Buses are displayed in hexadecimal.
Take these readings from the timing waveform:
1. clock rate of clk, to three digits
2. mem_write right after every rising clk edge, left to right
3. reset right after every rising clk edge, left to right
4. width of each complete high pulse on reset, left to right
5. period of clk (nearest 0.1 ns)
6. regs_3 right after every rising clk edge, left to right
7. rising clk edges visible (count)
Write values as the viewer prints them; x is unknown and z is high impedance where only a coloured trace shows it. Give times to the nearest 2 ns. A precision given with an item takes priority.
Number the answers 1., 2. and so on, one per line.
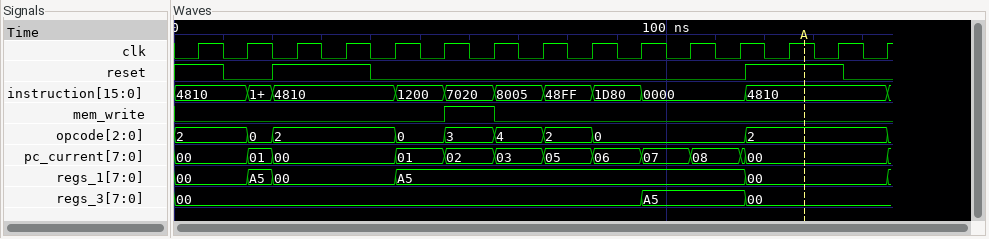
1. 100 MHz
2. 0 0 0 0 0 1 0 0 0 0 0 0 0 0 0
3. 1 0 1 1 0 0 0 0 0 0 0 0 1 1 0
4. 20 ns, 20 ns
5. 10 ns
6. 00, 00, 00, 00, 00, 00, 00, 00, 00, A5, A5, A5, 00, 00, 00
7. 15
